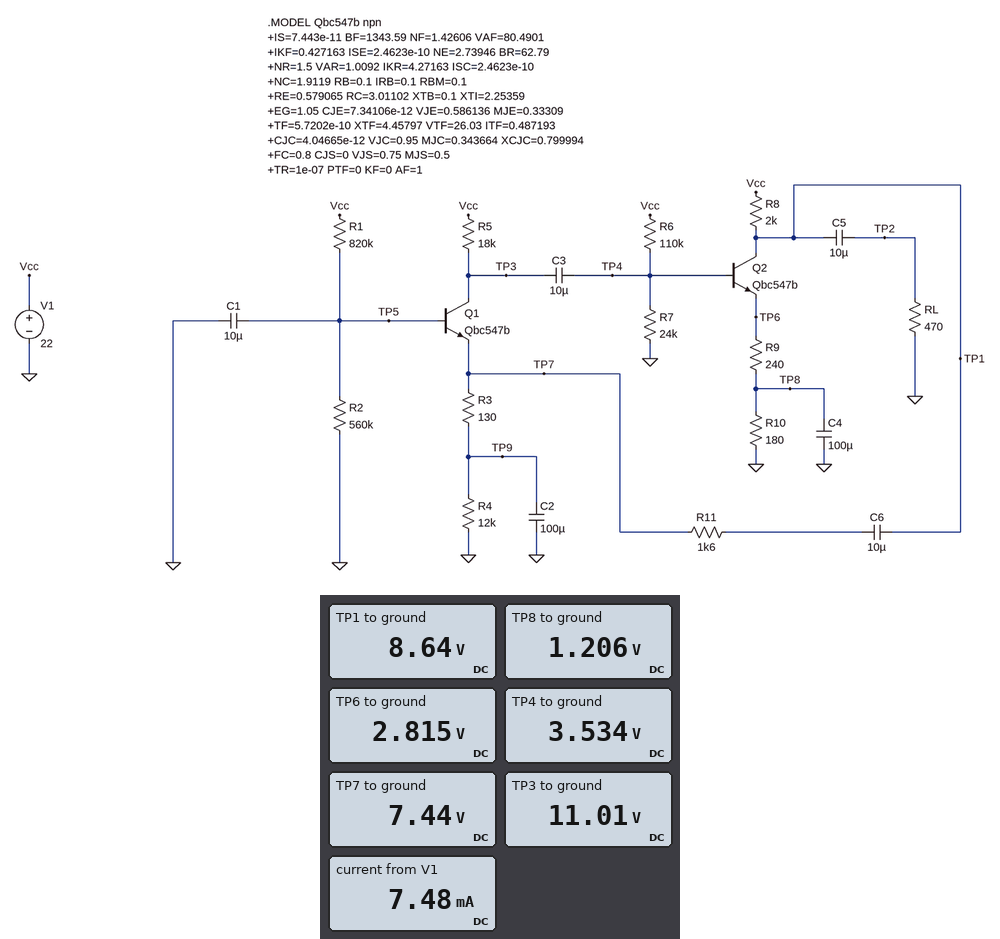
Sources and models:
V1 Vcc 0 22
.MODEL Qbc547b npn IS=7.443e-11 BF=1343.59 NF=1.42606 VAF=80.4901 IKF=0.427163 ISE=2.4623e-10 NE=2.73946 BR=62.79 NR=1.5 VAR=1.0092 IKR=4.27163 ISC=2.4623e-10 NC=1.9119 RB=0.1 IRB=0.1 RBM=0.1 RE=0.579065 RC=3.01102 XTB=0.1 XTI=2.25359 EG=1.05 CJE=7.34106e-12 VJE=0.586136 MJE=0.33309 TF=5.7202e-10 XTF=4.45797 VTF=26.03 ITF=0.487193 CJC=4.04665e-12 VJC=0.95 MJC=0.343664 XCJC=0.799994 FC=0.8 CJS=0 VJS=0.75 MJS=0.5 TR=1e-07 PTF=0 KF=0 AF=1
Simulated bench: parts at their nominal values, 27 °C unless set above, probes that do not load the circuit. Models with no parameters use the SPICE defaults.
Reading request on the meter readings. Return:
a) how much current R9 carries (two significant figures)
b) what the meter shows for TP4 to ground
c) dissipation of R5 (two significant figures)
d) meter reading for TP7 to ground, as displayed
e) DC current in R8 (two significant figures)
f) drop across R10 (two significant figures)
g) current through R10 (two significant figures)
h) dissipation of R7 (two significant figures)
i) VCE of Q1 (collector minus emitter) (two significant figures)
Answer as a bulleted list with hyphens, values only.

- 6.7 mA
- 3.534 V
- 6.7 mW
- 7.44 V
- 6.7 mA
- 1.2 V
- 6.7 mA
- 520 µW
- 3.6 V
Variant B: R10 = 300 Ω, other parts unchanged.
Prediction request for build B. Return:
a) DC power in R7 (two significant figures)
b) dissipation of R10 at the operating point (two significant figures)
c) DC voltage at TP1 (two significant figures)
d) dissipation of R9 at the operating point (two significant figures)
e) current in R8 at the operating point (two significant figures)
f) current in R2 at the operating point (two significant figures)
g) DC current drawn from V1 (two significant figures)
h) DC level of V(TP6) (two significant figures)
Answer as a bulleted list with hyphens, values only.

- 550 µW
- 8.8 mW
- 11 V
- 7.1 mW
- 5.4 mA
- 14 µA
- 6.2 mA
- 2.9 V
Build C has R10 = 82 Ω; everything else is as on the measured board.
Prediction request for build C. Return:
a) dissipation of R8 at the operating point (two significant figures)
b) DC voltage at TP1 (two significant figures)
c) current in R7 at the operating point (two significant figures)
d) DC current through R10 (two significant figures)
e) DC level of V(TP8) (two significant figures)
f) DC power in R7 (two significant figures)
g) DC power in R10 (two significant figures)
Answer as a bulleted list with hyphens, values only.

- 130 mW
- 5.6 V
- 140 µA
- 8.2 mA
- 670 mV
- 480 µW
- 5.5 mW
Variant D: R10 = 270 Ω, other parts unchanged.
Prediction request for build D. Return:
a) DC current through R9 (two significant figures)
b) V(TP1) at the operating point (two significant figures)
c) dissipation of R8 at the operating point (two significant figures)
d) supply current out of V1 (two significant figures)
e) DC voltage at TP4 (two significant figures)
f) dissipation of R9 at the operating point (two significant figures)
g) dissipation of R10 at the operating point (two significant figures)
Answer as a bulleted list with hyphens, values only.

- 5.7 mA
- 11 V
- 65 mW
- 6.5 mA
- 3.6 V
- 7.8 mW
- 8.8 mW
